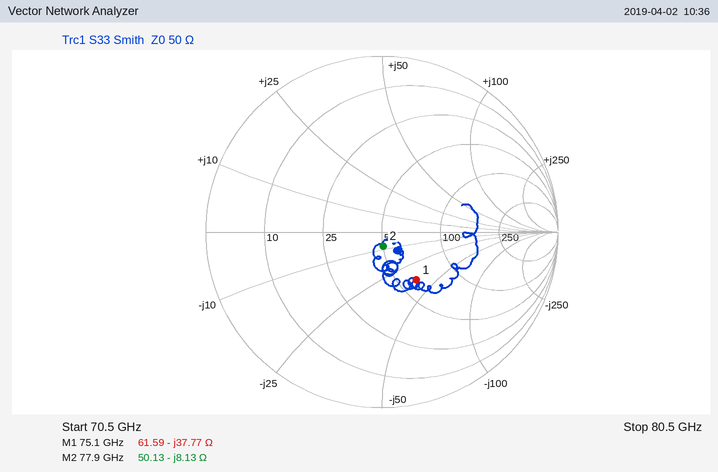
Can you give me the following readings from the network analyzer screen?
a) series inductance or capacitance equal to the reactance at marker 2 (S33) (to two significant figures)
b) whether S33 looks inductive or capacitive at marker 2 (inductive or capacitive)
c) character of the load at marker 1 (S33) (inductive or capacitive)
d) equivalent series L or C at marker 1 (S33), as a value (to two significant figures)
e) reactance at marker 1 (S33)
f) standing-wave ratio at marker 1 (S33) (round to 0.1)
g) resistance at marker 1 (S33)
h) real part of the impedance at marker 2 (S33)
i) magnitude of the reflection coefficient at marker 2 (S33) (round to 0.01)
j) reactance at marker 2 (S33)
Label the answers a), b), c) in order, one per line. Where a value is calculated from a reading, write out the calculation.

a) C = 1/(2π × 77.9 GHz × 8.13 Ω) ≈ 251 fF, so 250 fF to two significant figures
b) capacitive
c) capacitive
d) C = 1/(2π × 75.1 GHz × 37.77 Ω) ≈ 56 fF
e) -37.77 Ω
f) 2.0
g) 61.59 Ω
h) 50.13 Ω
i) 0.08
j) -8.13 Ω
